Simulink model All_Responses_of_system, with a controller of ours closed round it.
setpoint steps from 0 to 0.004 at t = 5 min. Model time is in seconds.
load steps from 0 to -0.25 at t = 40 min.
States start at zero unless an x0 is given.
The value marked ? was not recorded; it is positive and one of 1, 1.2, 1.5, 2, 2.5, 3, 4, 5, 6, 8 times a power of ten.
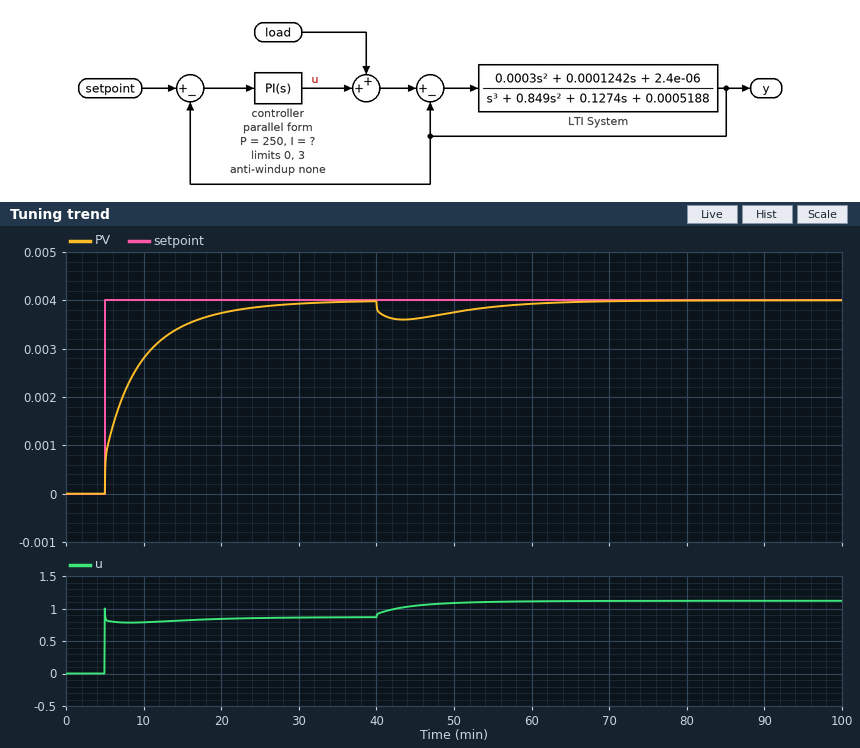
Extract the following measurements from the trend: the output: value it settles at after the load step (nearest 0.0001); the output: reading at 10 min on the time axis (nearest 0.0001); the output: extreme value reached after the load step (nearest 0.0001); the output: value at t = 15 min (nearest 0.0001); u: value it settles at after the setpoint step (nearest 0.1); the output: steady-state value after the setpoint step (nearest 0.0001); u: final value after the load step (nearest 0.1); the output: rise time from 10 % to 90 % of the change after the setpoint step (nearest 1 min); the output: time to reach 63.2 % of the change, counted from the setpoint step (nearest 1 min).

0.0040
0.0028
0.0036
0.0035
0.9
0.0040
1.1
12 min
4 min
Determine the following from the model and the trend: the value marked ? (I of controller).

0.8
